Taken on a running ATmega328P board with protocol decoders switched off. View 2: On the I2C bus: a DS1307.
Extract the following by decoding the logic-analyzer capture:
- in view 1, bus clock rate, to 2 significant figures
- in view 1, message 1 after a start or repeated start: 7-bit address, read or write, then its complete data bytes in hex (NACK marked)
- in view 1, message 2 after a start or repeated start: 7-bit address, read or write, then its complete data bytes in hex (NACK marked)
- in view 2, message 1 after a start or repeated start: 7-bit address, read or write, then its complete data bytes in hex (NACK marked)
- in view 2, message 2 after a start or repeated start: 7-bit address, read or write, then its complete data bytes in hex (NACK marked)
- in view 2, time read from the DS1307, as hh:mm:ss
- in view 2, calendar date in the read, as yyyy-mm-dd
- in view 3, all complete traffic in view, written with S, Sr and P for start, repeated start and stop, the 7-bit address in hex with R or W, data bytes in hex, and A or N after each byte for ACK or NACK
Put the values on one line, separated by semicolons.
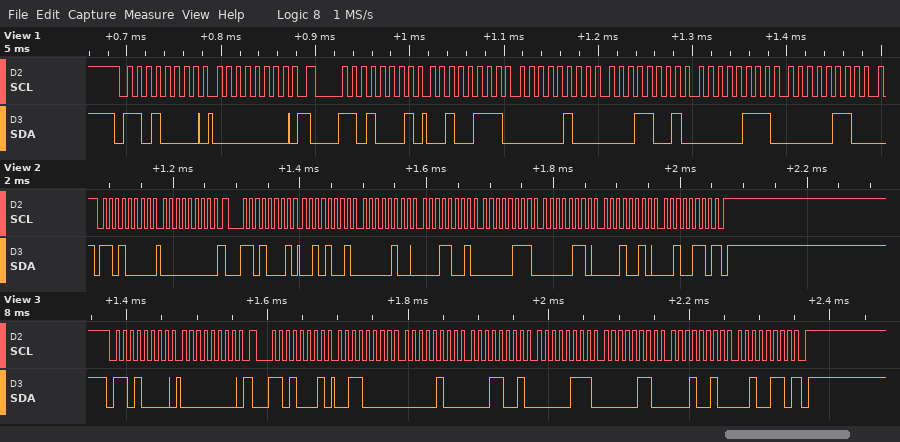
100 kHz; 0x68 write: 00; 0x68 read: 27 04 19 07 06; 0x68 write: 00; 0x68 read: 29 04 19 07 06 12 26 NACK; 19:04:29; 2026-12-06; S 68W A 00 A Sr 68R A 30 A 04 A 19 A 07 A 06 A 12 A 26 N P
